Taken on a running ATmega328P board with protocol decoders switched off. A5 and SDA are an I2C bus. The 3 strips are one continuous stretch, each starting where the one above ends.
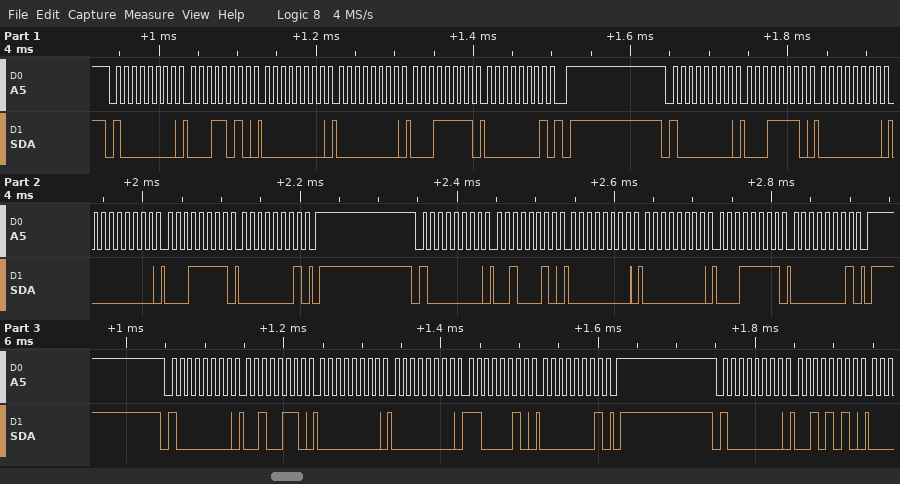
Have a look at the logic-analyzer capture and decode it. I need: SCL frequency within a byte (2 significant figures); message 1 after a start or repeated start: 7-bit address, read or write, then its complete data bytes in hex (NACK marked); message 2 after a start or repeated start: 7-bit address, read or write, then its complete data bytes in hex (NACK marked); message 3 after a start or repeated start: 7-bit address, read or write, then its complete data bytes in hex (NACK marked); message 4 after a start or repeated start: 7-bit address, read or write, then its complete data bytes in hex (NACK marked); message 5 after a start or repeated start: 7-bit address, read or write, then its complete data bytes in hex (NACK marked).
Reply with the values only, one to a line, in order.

100 kHz
0x40 write: 1A 00 00 1F 01
0x40 write: 1E 00 00 1F 01
0x40 write: 22 00 00 1F 01
0x40 write: 26 00 00 C2 01
0x40 write: 2A
